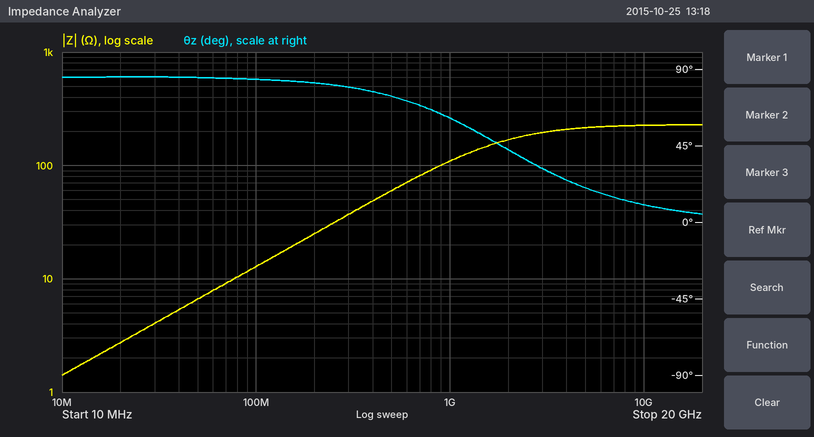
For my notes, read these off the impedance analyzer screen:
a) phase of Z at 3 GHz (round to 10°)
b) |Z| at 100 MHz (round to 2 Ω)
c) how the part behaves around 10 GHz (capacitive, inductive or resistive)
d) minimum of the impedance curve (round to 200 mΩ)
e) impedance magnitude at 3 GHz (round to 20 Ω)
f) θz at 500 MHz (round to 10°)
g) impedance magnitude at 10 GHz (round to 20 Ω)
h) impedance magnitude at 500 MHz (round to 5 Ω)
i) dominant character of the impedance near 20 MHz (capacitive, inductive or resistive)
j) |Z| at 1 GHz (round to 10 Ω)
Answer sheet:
30°
12 Ω
resistive
1.4 Ω
200 Ω
70°
220 Ω
60 Ω
inductive
110 Ω
